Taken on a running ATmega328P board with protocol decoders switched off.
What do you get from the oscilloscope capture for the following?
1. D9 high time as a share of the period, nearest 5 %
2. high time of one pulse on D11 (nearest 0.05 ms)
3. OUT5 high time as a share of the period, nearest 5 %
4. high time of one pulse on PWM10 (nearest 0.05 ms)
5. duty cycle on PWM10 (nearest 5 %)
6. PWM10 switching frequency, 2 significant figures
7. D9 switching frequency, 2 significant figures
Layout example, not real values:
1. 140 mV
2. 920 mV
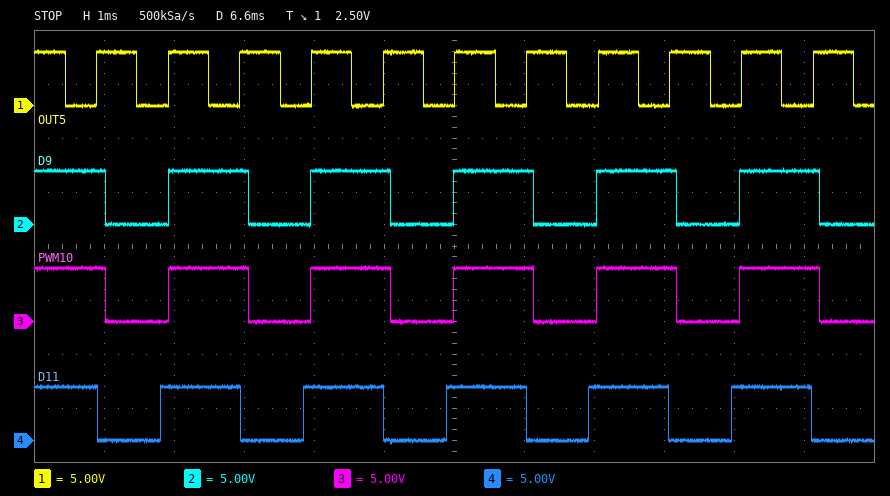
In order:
1. 55 %
2. 1.15 ms
3. 55 %
4. 1.15 ms
5. 55 %
6. 490 Hz
7. 490 Hz
